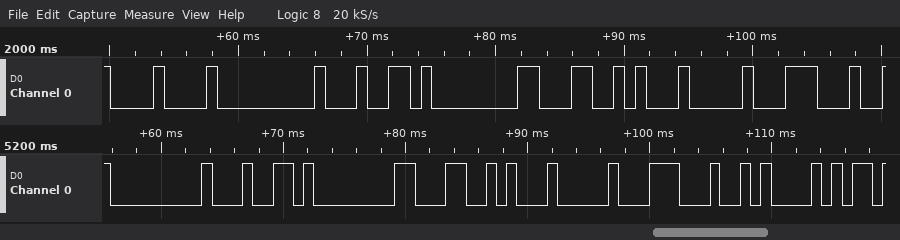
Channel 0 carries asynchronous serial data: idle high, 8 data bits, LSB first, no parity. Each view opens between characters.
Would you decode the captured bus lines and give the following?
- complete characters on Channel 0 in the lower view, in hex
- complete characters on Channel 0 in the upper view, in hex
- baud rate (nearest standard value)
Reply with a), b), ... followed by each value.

a) 00, 64, 80, 4C, 04, 1C, 0A
b) 08, 00, 64, 80, 4C, 04, 1C
c) 1200 baud
